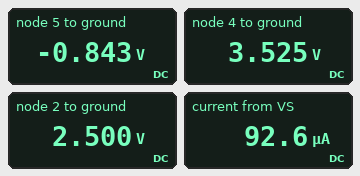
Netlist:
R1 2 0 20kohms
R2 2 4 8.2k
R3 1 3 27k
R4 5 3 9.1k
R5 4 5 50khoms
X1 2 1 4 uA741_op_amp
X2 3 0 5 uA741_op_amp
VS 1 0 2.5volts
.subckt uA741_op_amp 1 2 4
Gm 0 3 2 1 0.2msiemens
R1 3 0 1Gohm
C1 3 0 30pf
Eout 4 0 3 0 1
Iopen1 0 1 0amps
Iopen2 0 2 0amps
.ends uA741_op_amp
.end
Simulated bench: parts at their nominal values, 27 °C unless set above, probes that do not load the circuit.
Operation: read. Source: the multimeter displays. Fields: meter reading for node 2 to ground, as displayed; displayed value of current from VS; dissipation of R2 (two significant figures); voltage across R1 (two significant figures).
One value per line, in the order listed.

2.500 V
92.6 µA
130 µW
2.5 V
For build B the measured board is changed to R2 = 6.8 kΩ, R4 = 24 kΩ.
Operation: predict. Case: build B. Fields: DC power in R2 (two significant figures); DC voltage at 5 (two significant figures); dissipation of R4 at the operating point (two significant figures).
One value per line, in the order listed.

110 µW
-2.2 V
210 µW
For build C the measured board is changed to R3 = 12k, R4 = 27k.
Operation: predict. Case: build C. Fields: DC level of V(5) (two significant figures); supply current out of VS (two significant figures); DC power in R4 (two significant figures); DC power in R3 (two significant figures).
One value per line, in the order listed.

-5.6 V
210 µA
1.2 mW
520 µW
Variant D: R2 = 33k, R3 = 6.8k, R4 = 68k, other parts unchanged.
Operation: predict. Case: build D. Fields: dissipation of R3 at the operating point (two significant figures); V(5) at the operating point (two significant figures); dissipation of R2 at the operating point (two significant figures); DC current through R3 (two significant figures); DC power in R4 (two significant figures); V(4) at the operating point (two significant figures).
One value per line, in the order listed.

920 µW
-25 V
520 µW
370 µA
9.2 mW
6.6 V
